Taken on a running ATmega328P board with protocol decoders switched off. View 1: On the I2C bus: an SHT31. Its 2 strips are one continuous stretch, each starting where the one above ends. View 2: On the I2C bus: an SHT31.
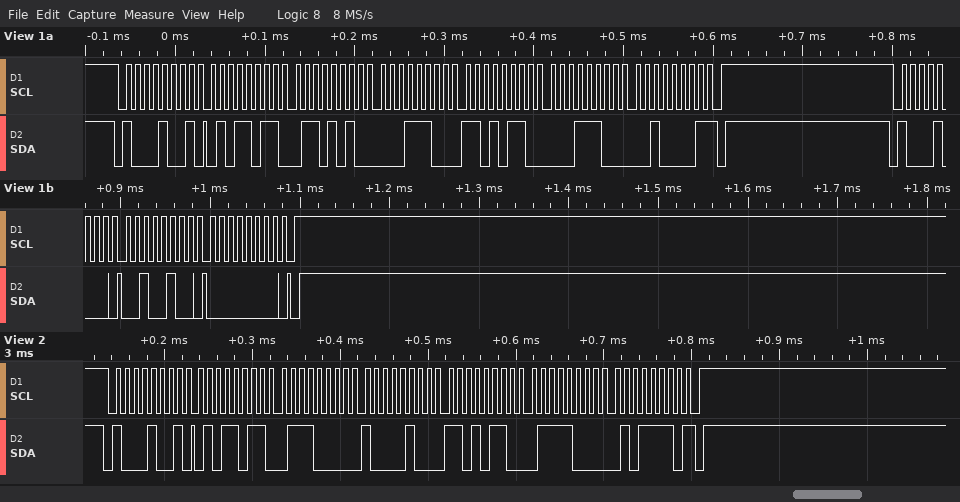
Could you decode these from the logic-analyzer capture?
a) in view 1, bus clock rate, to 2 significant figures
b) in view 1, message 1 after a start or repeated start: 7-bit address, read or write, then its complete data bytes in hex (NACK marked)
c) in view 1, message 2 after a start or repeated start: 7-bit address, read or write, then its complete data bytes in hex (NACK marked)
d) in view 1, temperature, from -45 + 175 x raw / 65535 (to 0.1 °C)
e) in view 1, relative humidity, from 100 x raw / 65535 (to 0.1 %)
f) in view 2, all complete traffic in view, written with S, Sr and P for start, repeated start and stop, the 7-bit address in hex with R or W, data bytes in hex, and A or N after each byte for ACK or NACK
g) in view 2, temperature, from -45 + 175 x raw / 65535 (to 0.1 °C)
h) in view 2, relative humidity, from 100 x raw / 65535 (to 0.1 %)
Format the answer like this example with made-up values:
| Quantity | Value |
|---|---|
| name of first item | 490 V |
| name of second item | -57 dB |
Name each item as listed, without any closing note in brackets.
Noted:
| Quantity | Value |
|---|---|
| in view 1, bus clock rate, to 2 significant figures | 100 kHz |
| in view 1, message 1 after a start or repeated start: 7-bit address, read or write, then its complete data bytes in hex | 0x44 read: 5B 6A 1C D6 1C 21 NACK |
| in view 1, message 2 after a start or repeated start: 7-bit address, read or write, then its complete data bytes in hex | 0x44 write: 24 00 |
| in view 1, temperature, from -45 + 175 x raw / 65535 | 17.5 °C |
| in view 1, relative humidity, from 100 x raw / 65535 | 83.6 % |
| in view 2, all complete traffic in view, written with S, Sr and P for start, repeated start and stop, the 7-bit address in hex with R or W, data bytes in hex, and A or N after each byte for ACK or NACK | S 44R A 5B A 70 A 84 A D6 A 78 A 5E N P |
| in view 2, temperature, from -45 + 175 x raw / 65535 | 17.5 °C |
| in view 2, relative humidity, from 100 x raw / 65535 | 83.8 % |
